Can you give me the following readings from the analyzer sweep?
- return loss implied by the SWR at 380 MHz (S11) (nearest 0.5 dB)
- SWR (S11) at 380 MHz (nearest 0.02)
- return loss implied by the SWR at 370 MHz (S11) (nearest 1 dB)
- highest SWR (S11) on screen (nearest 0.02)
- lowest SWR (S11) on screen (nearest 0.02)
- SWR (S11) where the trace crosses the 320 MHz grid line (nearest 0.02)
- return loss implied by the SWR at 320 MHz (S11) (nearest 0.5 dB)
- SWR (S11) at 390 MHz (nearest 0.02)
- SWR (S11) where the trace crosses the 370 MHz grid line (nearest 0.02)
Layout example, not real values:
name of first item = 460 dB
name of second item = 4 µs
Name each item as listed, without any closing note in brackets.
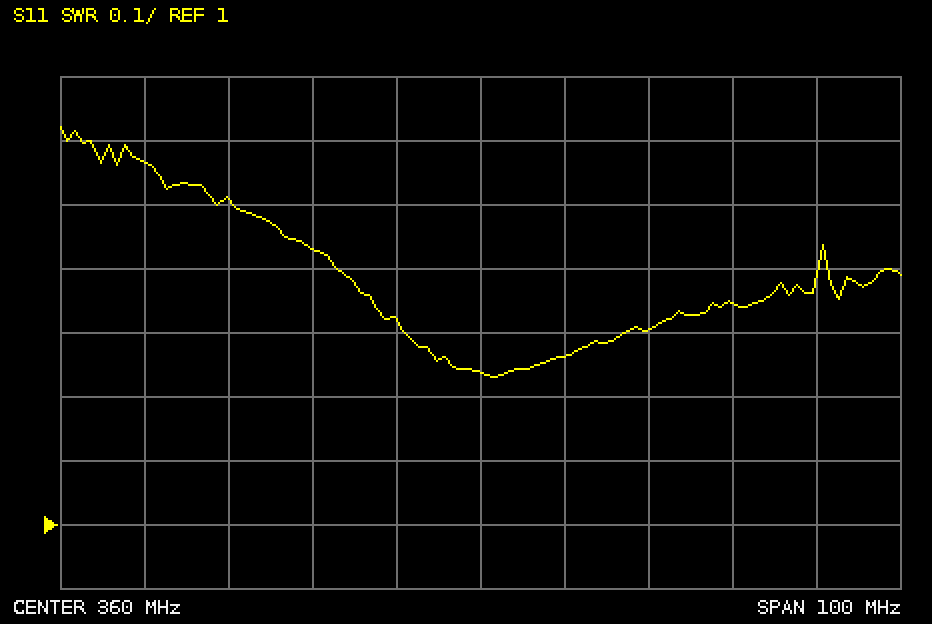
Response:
return loss implied by the SWR at 380 MHz (S11) = 17.5 dB
SWR (S11) at 380 MHz = 1.30
return loss implied by the SWR at 370 MHz (S11) = 19 dB
highest SWR (S11) on screen = 1.62
lowest SWR (S11) on screen = 1.24
SWR (S11) where the trace crosses the 320 MHz grid line = 1.56
return loss implied by the SWR at 320 MHz (S11) = 13.0 dB
SWR (S11) at 390 MHz = 1.34
SWR (S11) where the trace crosses the 370 MHz grid line = 1.26
